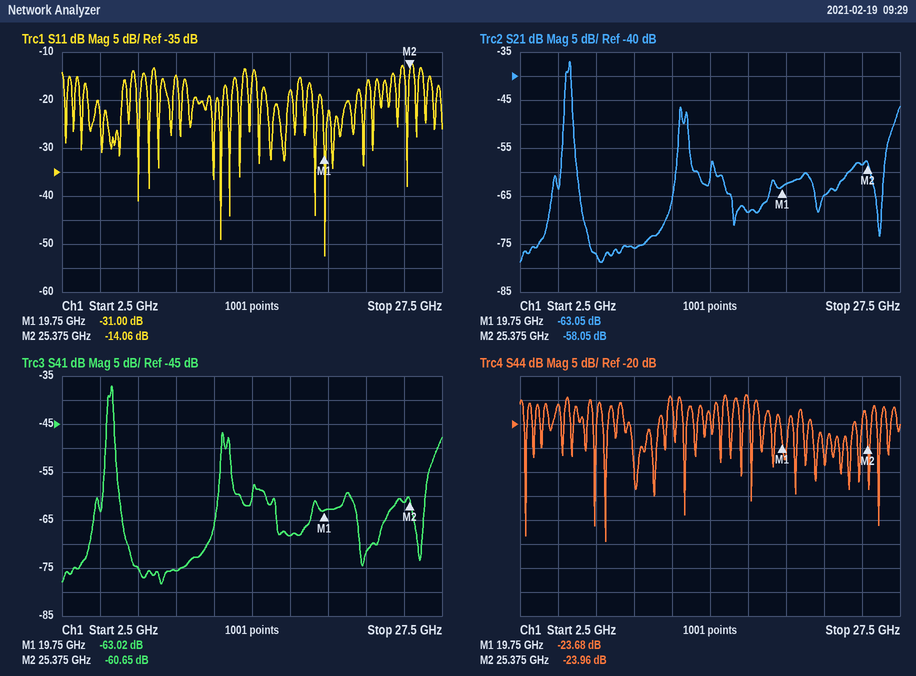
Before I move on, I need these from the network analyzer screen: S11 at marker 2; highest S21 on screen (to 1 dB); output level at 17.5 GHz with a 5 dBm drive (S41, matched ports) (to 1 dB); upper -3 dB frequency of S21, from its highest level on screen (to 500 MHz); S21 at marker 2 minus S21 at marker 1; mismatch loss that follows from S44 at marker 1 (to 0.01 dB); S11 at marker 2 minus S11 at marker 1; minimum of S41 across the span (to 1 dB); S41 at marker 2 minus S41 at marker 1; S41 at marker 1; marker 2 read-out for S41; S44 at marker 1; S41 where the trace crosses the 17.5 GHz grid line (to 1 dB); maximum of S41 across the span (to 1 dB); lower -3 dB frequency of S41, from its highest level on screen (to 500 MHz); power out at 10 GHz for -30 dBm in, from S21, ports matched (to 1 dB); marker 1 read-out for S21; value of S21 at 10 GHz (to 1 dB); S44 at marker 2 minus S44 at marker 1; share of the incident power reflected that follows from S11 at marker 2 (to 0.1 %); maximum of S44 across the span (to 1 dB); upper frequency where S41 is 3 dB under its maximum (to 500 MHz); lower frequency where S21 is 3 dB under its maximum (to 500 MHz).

-14.06 dB
-37 dB
-63 dBm
6.0 GHz
5.00 dB
0.02 dB
16.94 dB
-78 dB
2.37 dB
-63.02 dB
-60.65 dB
-23.68 dB
-68 dB
-37 dB
5.5 GHz
-106 dBm
-63.05 dB
-76 dB
-0.28 dB
3.9 %
-14 dB
6.0 GHz
5.5 GHz
